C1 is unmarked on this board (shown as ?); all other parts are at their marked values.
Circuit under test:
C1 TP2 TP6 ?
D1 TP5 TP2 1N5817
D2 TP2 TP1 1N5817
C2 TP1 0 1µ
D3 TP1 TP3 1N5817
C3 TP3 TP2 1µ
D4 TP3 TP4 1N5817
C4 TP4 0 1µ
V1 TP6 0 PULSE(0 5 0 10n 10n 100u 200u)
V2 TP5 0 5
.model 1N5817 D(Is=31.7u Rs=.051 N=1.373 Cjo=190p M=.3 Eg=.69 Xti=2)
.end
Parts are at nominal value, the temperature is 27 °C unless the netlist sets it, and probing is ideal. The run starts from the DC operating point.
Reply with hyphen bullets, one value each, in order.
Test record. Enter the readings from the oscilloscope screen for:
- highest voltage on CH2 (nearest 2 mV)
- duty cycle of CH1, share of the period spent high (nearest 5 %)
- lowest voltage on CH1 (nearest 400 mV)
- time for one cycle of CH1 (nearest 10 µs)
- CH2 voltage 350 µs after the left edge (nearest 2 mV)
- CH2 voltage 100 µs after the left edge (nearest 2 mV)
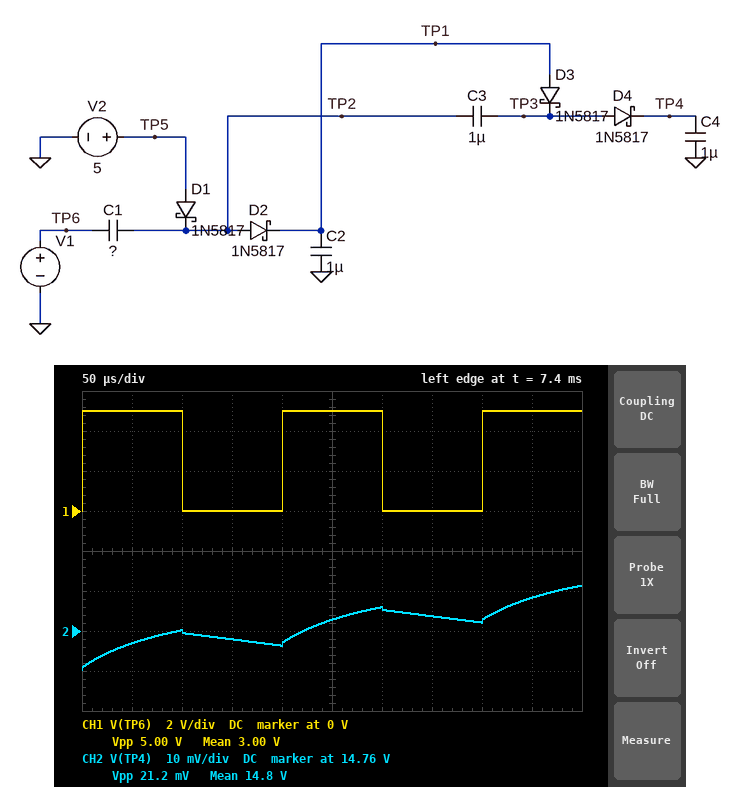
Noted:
- 14.772 V
- 50 %
- 0 V
- 200 µs
- 14.764 V
- 14.760 V
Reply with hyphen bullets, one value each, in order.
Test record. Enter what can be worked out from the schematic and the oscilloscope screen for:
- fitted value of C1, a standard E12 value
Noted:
- 2.7 µF
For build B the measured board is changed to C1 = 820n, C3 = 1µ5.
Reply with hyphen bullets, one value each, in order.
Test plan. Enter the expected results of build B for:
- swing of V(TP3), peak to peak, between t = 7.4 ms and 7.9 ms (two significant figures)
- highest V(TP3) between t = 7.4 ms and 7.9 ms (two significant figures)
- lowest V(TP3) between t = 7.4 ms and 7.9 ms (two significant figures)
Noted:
- 5.2 V
- 15 V
- 9.5 V
